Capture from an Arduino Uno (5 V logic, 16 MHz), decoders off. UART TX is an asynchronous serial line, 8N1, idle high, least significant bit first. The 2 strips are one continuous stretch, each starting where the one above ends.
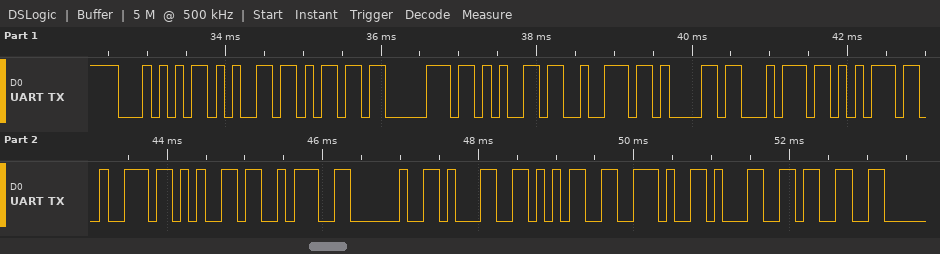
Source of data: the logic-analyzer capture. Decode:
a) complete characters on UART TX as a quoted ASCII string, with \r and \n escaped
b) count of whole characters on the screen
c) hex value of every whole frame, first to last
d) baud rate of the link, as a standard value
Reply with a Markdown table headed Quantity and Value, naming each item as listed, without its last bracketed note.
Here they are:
| Quantity | Value |
|---|---|
| complete characters on UART TX as a quoted ASCII string, with \r and \n escaped | "Temperature: 15.13" |
| count of whole characters on the screen | 18 |
| hex value of every whole frame, first to last | 54 65 6D 70 65 72 61 74 75 72 65 3A 20 31 35 2E 31 33 |
| baud rate of the link, as a standard value | 9600 baud |
